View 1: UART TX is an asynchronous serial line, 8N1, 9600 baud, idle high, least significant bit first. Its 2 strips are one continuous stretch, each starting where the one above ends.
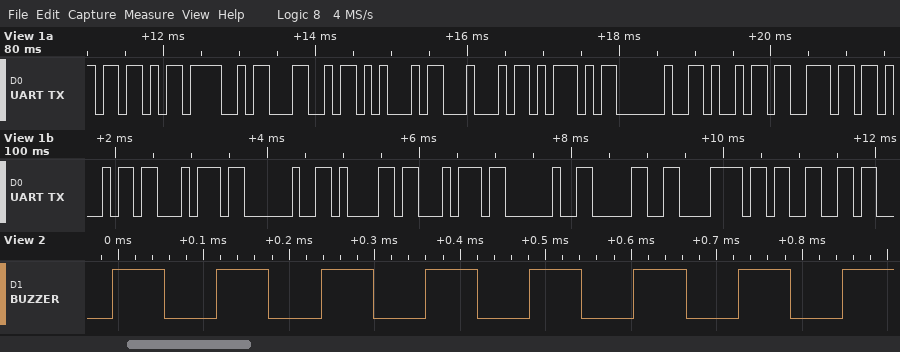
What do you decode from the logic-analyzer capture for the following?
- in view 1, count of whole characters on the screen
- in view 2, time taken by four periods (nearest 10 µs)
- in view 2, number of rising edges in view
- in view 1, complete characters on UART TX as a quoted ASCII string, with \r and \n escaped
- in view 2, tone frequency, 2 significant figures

18
490 µs
8
"[OLED] init at 0x3"
8.2 kHz
